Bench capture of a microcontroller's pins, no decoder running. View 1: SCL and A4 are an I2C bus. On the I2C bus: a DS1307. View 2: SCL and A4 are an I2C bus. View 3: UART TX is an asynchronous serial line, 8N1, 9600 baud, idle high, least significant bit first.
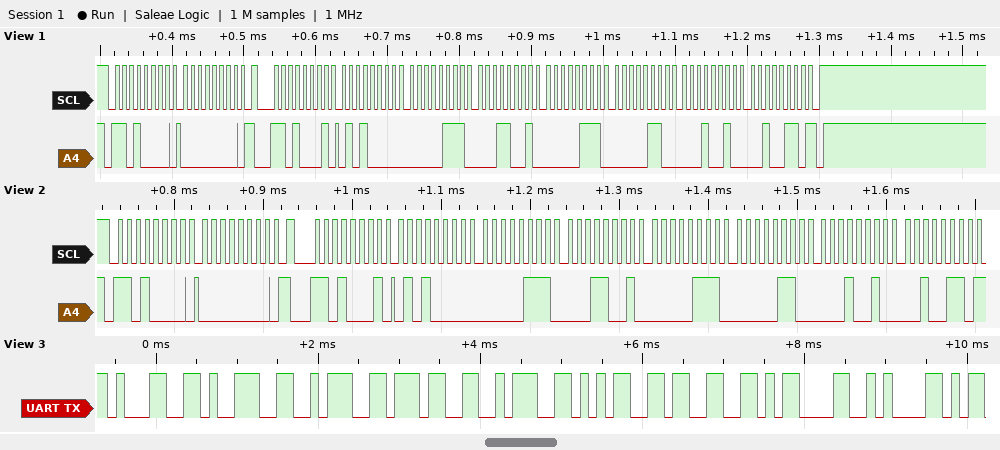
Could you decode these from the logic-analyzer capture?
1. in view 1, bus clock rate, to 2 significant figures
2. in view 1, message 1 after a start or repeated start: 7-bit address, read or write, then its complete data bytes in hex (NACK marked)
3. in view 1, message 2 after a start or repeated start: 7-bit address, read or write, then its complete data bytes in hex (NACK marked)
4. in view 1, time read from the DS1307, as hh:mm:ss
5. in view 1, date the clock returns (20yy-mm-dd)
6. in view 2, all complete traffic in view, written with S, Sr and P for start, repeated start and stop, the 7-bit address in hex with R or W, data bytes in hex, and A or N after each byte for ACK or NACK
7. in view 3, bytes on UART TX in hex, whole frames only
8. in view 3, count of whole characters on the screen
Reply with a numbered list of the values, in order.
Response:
1. 100 kHz
2. 0x68 write: 00
3. 0x68 read: 50 07 19 07 06 12 26 NACK
4. 19:07:50
5. 2026-12-06
6. S 68W A 00 A Sr 68R A 50 A 07 A 19 A 07 A 06 A 12 A 26 N
7. 31 39 3A 37 3A 35 33 0D 0A
8. 9
